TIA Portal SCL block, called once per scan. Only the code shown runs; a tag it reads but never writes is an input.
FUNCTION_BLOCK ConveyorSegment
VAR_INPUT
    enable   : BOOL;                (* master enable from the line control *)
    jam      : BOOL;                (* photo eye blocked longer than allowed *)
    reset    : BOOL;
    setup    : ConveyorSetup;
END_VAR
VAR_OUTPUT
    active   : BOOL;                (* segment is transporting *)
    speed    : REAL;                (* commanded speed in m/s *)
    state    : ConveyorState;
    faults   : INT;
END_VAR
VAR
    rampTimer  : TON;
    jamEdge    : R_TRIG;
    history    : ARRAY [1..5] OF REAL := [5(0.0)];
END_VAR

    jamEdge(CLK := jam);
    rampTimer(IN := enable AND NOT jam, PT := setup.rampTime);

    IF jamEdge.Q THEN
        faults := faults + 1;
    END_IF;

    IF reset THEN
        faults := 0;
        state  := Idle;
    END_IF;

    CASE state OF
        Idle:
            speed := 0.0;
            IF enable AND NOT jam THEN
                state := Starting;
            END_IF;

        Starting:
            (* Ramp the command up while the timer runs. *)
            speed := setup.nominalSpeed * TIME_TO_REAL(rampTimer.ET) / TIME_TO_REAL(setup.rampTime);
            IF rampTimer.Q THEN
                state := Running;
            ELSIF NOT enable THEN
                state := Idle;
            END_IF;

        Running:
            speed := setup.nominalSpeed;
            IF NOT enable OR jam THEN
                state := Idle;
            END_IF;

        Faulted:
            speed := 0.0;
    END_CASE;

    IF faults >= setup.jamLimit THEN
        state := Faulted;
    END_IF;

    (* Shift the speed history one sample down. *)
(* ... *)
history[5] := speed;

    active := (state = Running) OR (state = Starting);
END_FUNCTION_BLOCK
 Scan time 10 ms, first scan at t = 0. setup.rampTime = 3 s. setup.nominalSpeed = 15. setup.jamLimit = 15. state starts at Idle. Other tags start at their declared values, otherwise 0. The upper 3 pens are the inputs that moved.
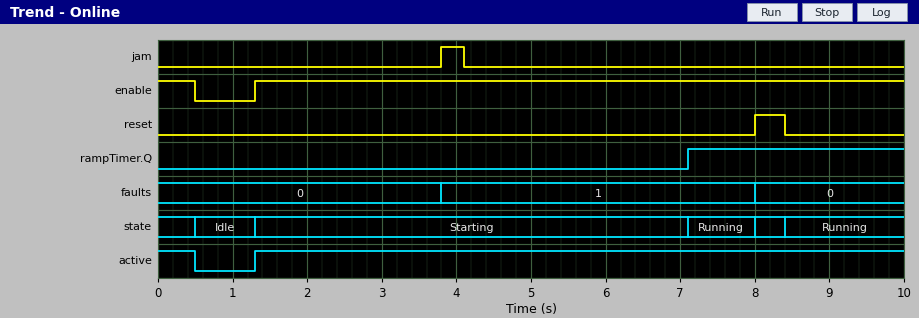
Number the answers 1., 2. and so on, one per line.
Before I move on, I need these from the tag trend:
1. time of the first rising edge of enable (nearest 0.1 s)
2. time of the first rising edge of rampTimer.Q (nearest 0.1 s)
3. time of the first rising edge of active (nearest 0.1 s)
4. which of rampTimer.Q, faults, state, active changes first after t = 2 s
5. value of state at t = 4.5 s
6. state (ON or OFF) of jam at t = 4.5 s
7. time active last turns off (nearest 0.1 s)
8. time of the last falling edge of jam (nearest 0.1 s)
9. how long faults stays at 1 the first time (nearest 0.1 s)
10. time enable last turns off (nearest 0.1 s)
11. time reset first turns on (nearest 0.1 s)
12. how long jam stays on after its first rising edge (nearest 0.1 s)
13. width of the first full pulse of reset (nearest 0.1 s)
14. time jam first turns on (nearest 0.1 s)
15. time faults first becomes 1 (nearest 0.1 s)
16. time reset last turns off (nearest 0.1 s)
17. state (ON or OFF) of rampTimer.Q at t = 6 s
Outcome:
1. 1.3 s
2. 7.1 s
3. 1.3 s
4. faults
5. Starting
6. OFF
7. 0.5 s
8. 4.1 s
9. 4.2 s
10. 0.5 s
11. 8.0 s
12. 0.3 s
13. 0.4 s
14. 3.8 s
15. 3.8 s
16. 8.4 s
17. OFF
